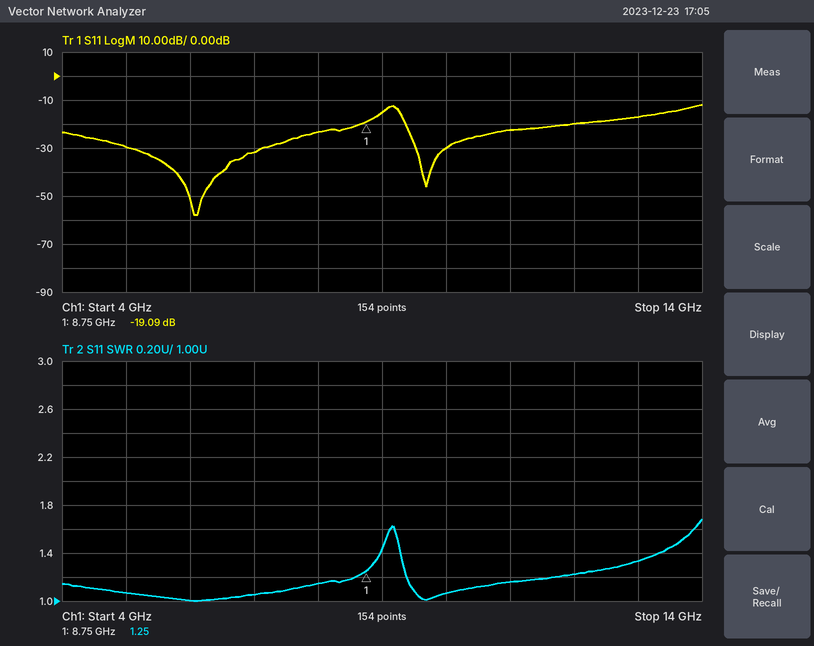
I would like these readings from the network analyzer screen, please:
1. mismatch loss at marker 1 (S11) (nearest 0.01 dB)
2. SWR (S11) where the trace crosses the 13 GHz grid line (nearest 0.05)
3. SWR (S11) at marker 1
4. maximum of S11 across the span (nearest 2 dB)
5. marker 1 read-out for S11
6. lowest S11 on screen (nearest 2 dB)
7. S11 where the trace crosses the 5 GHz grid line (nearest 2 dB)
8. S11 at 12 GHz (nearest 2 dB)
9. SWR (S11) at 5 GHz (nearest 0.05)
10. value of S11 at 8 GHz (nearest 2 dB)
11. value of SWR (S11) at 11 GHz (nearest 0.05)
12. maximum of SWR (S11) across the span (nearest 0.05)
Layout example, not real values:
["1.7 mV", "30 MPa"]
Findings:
["0.05 dB", "1.35", "1.25", "-12 dB", "-19.09 dB", "-58 dB", "-30 dB", "-20 dB", "1.05", "-24 dB", "1.15", "1.70"]
